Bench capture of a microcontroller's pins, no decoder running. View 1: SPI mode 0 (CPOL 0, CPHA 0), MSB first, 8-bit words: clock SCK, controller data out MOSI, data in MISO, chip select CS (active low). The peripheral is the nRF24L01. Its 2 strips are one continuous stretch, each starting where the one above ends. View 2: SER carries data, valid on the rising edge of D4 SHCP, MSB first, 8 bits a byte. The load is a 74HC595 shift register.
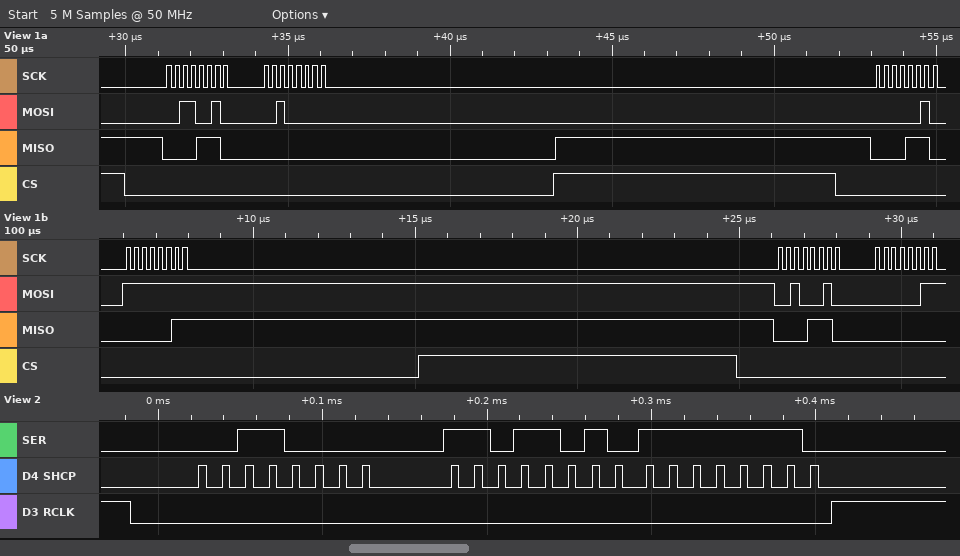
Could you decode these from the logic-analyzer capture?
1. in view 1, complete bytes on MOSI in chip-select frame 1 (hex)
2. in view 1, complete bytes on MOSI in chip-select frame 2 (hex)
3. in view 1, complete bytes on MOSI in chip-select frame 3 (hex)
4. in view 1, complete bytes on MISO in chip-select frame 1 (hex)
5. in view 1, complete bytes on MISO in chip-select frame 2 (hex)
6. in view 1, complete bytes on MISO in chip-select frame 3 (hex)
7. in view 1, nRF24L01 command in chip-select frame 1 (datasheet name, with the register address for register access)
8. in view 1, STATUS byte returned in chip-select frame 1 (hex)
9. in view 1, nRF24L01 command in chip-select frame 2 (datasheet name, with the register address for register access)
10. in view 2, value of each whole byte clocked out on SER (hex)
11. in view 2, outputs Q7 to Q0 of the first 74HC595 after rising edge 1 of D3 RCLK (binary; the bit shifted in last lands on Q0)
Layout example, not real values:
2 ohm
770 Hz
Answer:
32 20
02 FF
22 03
0E 00
0E 03
0E 00
W_REGISTER 0x12
0x0E
R_REGISTER 0x02
30 DA FE
11111110
